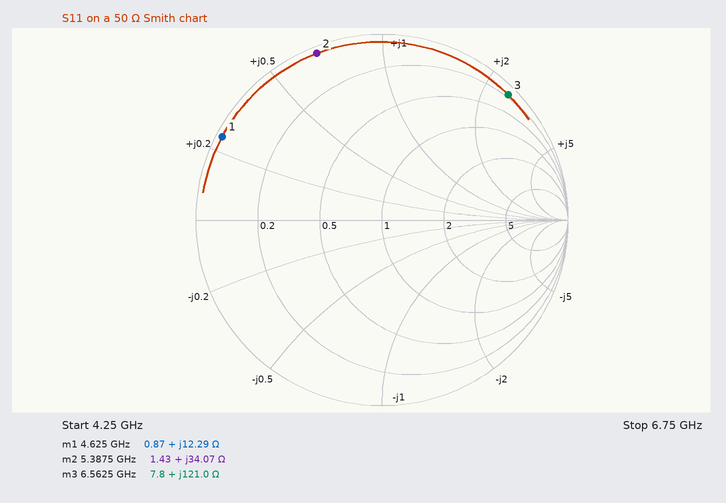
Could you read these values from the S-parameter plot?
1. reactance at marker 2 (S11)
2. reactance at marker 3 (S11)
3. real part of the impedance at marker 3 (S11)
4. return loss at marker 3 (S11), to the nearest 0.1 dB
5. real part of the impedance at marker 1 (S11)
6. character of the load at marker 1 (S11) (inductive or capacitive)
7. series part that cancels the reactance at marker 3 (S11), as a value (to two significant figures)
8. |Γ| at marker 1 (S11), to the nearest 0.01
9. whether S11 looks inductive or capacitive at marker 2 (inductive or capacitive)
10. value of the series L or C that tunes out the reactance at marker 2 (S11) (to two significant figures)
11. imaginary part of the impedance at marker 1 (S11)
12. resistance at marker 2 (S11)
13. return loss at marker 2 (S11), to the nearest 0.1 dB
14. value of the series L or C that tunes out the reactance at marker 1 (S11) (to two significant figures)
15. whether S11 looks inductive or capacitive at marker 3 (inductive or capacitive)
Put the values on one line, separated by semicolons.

+34.07 Ω; +121.0 Ω; 7.8 Ω; 0.4 dB; 0.87 Ω; inductive; 200 fF; 0.97; inductive; 870 fF; +12.29 Ω; 1.43 Ω; 0.3 dB; 2.8 pF; inductive
